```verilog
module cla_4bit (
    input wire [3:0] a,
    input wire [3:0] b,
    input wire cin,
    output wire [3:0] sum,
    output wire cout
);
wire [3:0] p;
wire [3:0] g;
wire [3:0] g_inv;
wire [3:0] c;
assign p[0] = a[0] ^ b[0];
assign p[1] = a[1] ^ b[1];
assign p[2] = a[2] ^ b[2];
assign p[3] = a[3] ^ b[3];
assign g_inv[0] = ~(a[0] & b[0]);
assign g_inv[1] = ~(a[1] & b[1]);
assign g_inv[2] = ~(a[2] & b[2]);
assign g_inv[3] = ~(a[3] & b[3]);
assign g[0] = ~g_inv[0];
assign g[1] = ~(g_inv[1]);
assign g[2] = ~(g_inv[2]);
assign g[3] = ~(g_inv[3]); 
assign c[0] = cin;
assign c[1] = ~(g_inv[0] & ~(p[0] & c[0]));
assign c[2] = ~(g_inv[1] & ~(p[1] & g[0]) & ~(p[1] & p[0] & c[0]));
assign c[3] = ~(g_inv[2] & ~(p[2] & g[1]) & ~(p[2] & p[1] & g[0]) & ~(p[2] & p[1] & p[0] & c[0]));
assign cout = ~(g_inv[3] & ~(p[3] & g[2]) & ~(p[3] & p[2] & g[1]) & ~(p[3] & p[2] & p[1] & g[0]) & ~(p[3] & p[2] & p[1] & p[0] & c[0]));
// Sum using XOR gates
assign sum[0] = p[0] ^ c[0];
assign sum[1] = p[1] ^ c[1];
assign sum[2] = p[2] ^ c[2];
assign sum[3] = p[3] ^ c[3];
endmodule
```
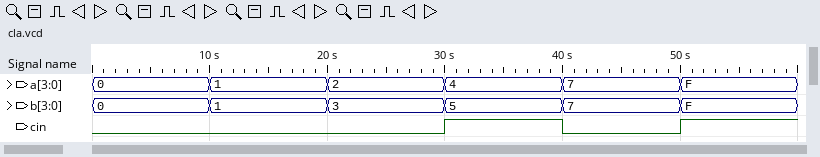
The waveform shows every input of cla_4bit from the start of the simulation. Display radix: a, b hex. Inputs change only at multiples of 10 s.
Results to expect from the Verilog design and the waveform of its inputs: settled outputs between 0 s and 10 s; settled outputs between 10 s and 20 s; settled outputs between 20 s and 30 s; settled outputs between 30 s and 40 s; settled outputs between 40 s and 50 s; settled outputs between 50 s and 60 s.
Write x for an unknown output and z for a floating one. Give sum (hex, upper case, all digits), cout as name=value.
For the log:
sum=0, cout=0
sum=2, cout=0
sum=5, cout=0
sum=A, cout=0
sum=E, cout=0
sum=F, cout=1
